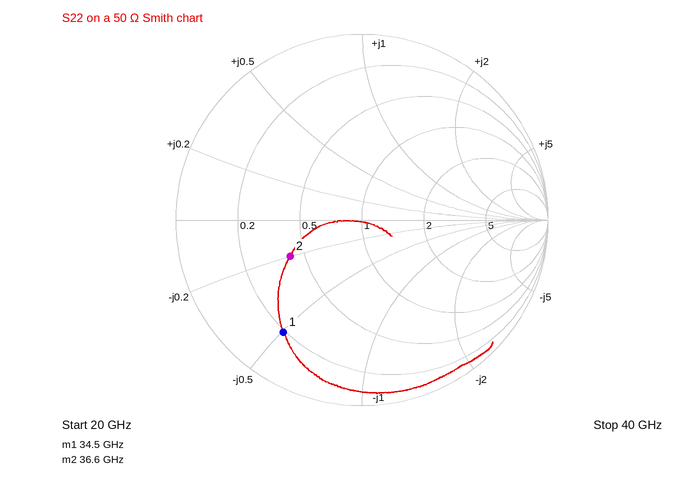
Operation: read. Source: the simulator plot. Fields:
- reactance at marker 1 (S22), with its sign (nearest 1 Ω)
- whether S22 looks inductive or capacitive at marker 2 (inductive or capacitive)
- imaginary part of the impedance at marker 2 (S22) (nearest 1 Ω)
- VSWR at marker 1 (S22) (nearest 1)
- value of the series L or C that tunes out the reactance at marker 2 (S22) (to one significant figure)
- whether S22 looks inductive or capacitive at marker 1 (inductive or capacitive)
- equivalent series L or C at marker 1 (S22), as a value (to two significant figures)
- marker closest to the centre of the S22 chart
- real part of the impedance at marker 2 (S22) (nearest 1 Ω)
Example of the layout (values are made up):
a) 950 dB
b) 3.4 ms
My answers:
a) -25 Ω
b) capacitive
c) -10 Ω
d) 7
e) 40 pH
f) capacitive
g) 180 fF
h) marker 2
i) 21 Ω
